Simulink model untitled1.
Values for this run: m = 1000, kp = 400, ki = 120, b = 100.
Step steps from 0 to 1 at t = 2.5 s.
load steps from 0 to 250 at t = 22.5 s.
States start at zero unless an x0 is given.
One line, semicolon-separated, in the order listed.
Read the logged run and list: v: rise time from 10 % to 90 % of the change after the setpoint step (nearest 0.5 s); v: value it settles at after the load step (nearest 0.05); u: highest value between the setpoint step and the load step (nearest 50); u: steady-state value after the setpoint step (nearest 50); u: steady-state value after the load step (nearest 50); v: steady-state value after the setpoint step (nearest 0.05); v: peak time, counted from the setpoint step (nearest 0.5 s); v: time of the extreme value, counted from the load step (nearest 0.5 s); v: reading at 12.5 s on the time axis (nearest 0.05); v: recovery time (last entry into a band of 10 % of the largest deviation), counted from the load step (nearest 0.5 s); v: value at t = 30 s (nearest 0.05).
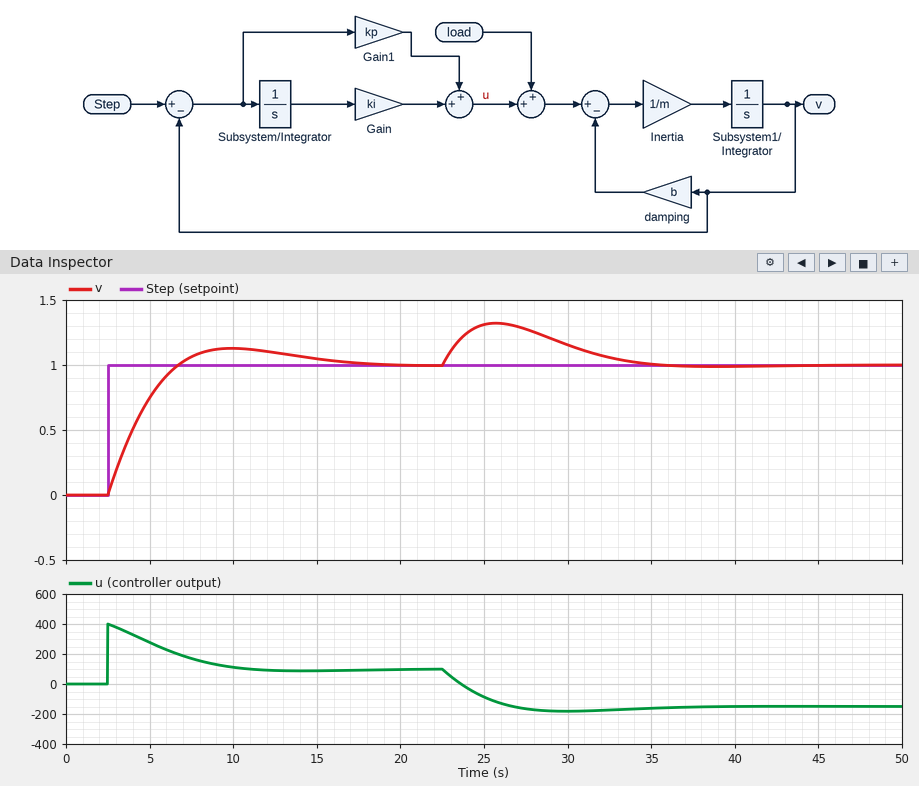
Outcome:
3.0 s; 1.00; 400; 100; -150; 1.00; 7.5 s; 3.0 s; 1.10; 11.0 s; 1.15
